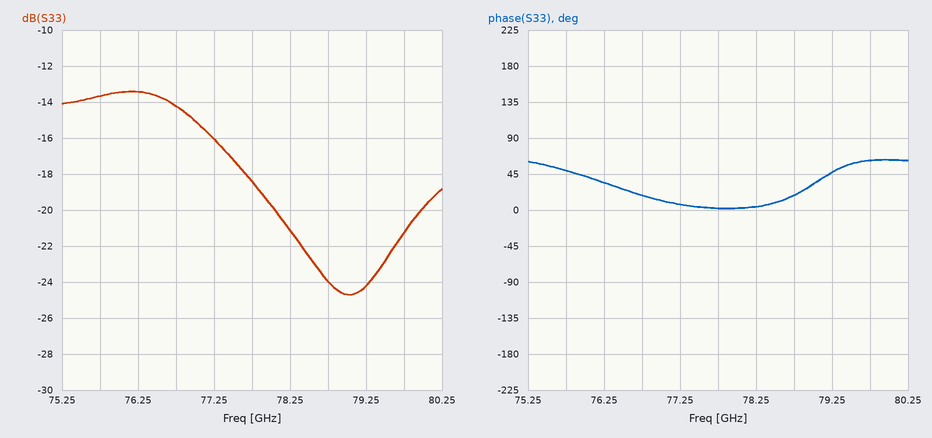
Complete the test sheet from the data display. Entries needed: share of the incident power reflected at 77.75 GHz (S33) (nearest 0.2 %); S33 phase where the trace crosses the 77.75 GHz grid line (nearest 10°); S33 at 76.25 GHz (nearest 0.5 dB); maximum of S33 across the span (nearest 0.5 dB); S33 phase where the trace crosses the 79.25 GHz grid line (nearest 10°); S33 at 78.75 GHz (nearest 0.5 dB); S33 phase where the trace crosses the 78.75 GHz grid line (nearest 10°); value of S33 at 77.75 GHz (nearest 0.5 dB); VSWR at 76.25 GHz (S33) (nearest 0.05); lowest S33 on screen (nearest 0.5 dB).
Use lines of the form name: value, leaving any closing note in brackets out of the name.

share of the incident power reflected at 77.75 GHz (S33): 1.4 %
S33 phase where the trace crosses the 77.75 GHz grid line: 0°
S33 at 76.25 GHz: -13.5 dB
maximum of S33 across the span: -13.5 dB
S33 phase where the trace crosses the 79.25 GHz grid line: 50°
S33 at 78.75 GHz: -24.0 dB
S33 phase where the trace crosses the 78.75 GHz grid line: 20°
value of S33 at 77.75 GHz: -18.5 dB
VSWR at 76.25 GHz (S33): 1.55
lowest S33 on screen: -24.5 dB
